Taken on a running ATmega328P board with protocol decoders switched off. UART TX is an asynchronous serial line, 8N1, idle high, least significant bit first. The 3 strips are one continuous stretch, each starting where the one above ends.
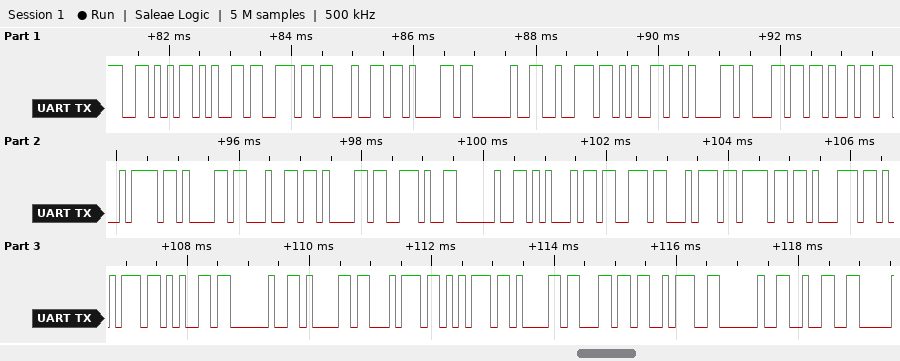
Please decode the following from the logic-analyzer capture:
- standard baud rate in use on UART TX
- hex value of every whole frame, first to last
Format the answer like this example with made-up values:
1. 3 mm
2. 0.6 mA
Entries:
1. 9600 baud
2. 56 65 6E 64 61 20 72 65 61 6C 69 7A 61 64 61 2E 20 45 73 74 6F 71 75 65 20 61 74 75 61 6C 3A 20 32
